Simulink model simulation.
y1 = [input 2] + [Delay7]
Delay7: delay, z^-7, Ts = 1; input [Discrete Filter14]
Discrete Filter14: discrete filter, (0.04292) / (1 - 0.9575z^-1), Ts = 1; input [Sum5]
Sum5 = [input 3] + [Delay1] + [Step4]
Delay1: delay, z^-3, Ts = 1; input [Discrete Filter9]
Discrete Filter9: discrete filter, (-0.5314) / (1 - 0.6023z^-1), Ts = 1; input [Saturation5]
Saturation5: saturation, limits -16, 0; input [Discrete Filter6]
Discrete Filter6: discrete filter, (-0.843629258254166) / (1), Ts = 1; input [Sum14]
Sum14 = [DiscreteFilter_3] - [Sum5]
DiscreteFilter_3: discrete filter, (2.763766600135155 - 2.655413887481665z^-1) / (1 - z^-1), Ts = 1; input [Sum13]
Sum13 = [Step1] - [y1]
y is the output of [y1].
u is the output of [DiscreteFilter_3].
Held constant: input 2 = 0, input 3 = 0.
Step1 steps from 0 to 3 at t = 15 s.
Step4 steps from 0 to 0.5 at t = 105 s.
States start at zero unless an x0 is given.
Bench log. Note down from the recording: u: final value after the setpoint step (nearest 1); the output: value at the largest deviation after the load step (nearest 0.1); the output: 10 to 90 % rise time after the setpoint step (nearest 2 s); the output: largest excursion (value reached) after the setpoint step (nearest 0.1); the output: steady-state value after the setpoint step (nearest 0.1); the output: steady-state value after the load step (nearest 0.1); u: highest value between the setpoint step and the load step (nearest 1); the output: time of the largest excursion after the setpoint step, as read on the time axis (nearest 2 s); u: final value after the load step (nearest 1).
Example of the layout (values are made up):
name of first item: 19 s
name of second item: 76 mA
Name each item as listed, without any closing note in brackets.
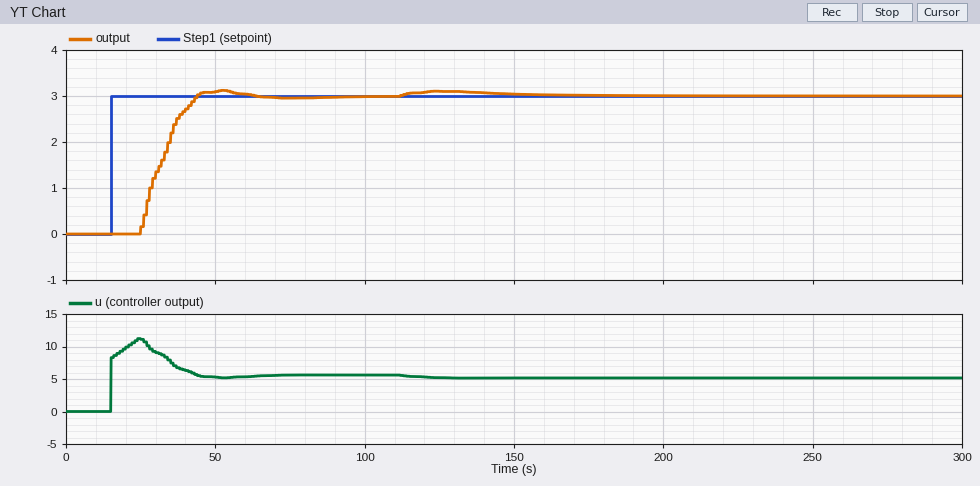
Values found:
u: final value after the setpoint step: 6
the output: value at the largest deviation after the load step: 3.1
the output: 10 to 90 % rise time after the setpoint step: 14 s
the output: largest excursion (value reached) after the setpoint step: 3.1
the output: steady-state value after the setpoint step: 3.0
the output: steady-state value after the load step: 3.0
u: highest value between the setpoint step and the load step: 11
the output: time of the largest excursion after the setpoint step, as read on the time axis: 52 s
u: final value after the load step: 5
